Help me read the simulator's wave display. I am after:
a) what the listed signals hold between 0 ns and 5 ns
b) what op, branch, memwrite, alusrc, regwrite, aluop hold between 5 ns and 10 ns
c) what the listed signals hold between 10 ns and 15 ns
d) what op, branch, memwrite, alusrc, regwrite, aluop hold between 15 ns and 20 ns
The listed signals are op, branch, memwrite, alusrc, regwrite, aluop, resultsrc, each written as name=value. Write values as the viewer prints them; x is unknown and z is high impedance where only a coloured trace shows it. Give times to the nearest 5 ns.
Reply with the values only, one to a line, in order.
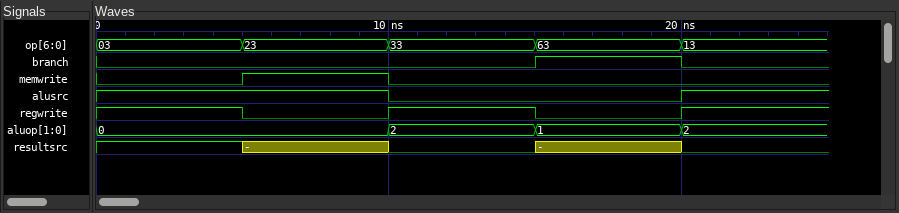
op=03, branch=0, memwrite=0, alusrc=1, regwrite=1, aluop=0, resultsrc=1
op=23, branch=0, memwrite=1, alusrc=1, regwrite=0, aluop=0
op=33, branch=0, memwrite=0, alusrc=0, regwrite=1, aluop=2, resultsrc=0
op=63, branch=1, memwrite=0, alusrc=0, regwrite=0, aluop=1
